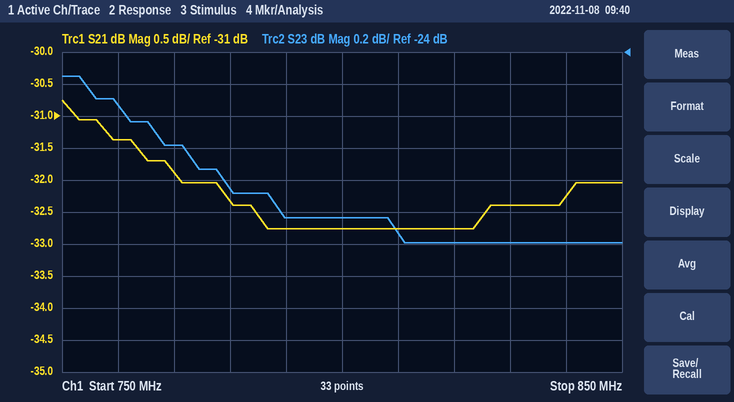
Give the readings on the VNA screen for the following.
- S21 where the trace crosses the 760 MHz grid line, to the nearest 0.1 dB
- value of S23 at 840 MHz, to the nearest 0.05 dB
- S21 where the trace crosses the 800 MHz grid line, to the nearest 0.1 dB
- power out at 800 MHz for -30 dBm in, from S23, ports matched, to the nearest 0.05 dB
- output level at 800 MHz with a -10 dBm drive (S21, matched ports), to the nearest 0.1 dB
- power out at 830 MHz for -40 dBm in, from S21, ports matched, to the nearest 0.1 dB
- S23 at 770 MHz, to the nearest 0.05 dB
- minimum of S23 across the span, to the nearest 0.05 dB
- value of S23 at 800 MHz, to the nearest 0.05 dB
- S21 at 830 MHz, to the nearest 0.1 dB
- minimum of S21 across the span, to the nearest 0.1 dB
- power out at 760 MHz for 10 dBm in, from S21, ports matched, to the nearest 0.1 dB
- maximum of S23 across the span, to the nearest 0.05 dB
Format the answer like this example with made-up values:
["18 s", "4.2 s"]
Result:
["-31.4 dB", "-25.20 dB", "-32.8 dB", "-55.05 dBm", "-42.8 dBm", "-72.4 dBm", "-24.60 dB", "-25.20 dB", "-25.05 dB", "-32.4 dB", "-32.8 dB", "-21.4 dBm", "-24.15 dB"]
